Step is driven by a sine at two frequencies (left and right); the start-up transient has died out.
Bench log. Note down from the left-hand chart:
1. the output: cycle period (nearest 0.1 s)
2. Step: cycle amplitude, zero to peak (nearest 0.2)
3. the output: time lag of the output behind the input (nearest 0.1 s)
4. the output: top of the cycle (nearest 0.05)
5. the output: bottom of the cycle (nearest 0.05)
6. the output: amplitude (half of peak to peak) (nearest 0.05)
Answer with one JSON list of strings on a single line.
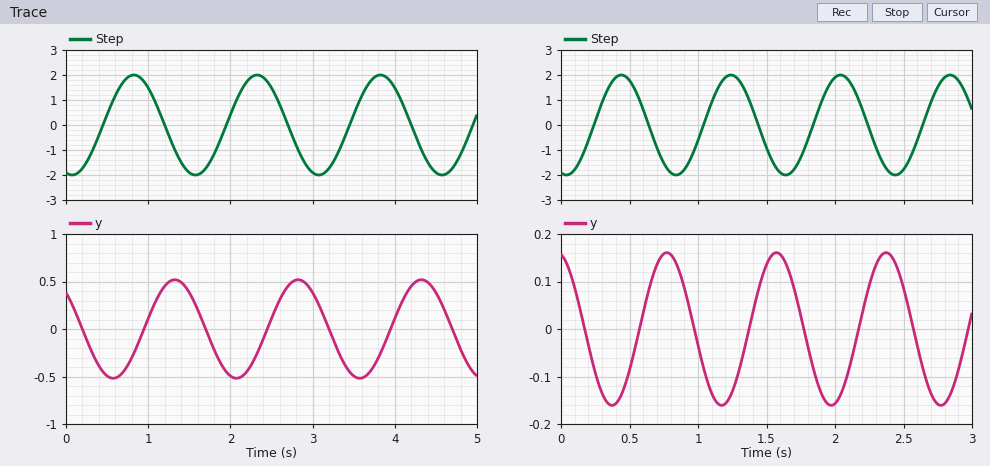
["1.5 s", "2.0", "0.5 s", "0.50", "-0.50", "0.50"]
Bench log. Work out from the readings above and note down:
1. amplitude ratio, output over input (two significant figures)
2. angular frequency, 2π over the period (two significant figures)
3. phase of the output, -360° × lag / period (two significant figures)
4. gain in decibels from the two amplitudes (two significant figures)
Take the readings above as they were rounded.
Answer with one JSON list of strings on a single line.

["0.25", "4.2 rad/s", "-120°", "-12 dB"]
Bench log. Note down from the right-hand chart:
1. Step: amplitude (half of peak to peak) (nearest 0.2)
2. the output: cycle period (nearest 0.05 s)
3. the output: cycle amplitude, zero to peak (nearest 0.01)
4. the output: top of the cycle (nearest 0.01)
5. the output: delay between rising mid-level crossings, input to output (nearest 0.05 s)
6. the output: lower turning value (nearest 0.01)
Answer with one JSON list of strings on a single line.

["2.0", "0.80 s", "0.16", "0.16", "0.35 s", "-0.16"]
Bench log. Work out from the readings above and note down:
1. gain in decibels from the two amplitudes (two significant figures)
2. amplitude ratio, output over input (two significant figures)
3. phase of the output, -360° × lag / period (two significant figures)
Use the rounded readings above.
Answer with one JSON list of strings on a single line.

["-22 dB", "0.080", "-160°"]
